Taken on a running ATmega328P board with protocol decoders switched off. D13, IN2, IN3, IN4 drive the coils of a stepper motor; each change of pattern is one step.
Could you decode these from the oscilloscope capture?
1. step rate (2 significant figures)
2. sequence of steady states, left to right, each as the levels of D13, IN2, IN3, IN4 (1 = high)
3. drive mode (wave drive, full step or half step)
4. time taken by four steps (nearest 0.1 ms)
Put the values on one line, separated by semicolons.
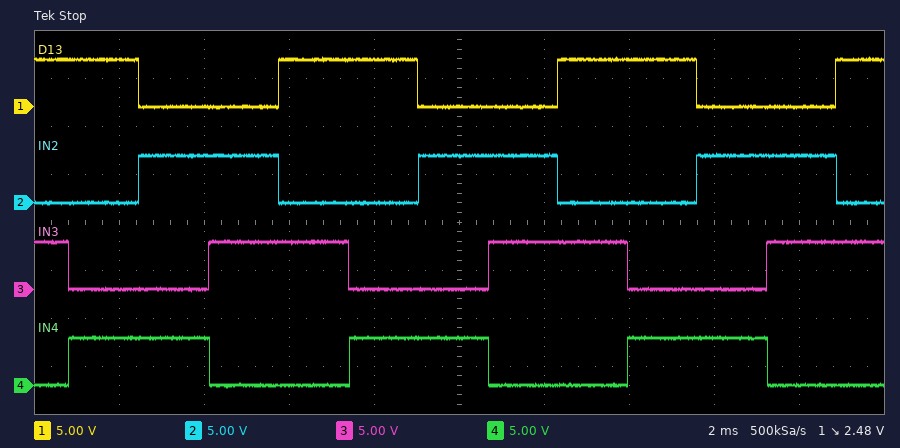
610 steps/s; 1010 1001 0101 0110 1010 1001 0101 0110 1010 1001 0101 0110 1010; full step; 6.6 ms
